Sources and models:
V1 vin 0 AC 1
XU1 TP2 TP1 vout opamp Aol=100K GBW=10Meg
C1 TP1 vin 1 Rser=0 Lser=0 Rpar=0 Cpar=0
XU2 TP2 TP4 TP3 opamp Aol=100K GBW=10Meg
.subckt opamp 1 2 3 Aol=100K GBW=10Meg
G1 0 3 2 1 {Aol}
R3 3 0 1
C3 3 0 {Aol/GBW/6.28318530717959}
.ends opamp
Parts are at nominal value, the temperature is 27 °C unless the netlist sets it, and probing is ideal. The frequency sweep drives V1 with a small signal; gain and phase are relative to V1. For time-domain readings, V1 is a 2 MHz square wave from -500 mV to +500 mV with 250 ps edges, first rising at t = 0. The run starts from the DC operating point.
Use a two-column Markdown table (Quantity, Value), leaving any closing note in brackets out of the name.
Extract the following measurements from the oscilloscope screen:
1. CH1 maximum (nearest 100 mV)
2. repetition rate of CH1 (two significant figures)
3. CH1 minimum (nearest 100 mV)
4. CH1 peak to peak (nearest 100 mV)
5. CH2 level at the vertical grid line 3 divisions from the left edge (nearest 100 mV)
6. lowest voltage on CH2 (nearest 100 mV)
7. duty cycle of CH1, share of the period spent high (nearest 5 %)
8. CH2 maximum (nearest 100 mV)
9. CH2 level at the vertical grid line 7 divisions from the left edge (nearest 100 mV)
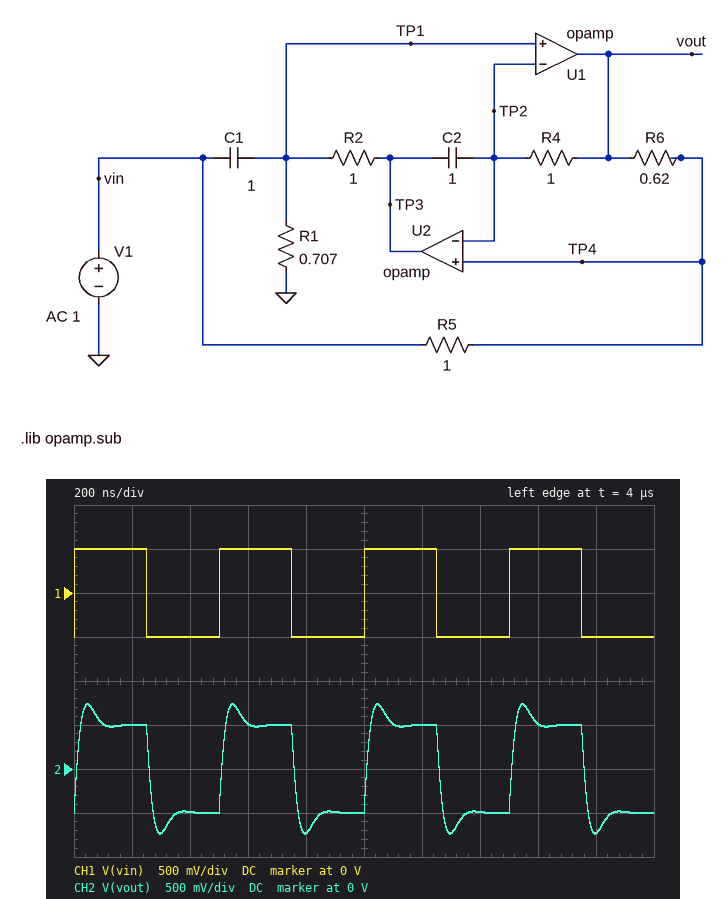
| Quantity | Value |
|---|---|
| CH1 maximum | 500 mV |
| repetition rate of CH1 | 2.0 MHz |
| CH1 minimum | -500 mV |
| CH1 peak to peak | 1.0 V |
| CH2 level at the vertical grid line 3 divisions from the left edge | 500 mV |
| lowest voltage on CH2 | -700 mV |
| duty cycle of CH1, share of the period spent high | 50 % |
| CH2 maximum | 700 mV |
| CH2 level at the vertical grid line 7 divisions from the left edge | -500 mV |
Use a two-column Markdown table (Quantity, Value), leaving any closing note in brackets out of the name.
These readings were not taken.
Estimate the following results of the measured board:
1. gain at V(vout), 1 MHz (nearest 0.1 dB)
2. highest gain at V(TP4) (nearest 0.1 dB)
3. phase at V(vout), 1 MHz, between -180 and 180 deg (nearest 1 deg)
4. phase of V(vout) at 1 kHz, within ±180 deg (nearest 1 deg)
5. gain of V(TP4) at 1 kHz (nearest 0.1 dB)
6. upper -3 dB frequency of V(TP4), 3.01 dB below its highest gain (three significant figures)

| Quantity | Value |
|---|---|
| gain at V(vout), 1 MHz | 0.1 dB |
| highest gain at V(TP4) | 1.4 dB |
| phase at V(vout), 1 MHz, between -180 and 180 deg | 0 deg |
| phase of V(vout) at 1 kHz, within ±180 deg | 0 deg |
| gain of V(TP4) at 1 kHz | 0 dB |
| upper -3 dB frequency of V(TP4), 3.01 dB below its highest gain | 11.9 MHz |
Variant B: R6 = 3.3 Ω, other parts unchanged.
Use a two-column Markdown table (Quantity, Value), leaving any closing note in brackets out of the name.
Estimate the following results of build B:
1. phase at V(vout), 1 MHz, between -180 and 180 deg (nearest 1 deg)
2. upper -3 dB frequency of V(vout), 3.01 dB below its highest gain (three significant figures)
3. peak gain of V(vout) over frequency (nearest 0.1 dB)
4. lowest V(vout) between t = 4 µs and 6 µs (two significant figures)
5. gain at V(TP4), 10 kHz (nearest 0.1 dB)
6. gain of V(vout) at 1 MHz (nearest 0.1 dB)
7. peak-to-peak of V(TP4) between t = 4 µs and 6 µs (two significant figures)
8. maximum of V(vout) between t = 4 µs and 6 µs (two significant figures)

| Quantity | Value |
|---|---|
| phase at V(vout), 1 MHz, between -180 and 180 deg | -1 deg |
| upper -3 dB frequency of V(vout), 3.01 dB below its highest gain | 439 mHz |
| peak gain of V(vout) over frequency | 10.4 dB |
| lowest V(vout) between t = 4 µs and 6 µs | -630 mV |
| gain at V(TP4), 10 kHz | 0 dB |
| gain of V(vout) at 1 MHz | 0.3 dB |
| peak-to-peak of V(TP4) between t = 4 µs and 6 µs | 1.1 V |
| maximum of V(vout) between t = 4 µs and 6 µs | 630 mV |
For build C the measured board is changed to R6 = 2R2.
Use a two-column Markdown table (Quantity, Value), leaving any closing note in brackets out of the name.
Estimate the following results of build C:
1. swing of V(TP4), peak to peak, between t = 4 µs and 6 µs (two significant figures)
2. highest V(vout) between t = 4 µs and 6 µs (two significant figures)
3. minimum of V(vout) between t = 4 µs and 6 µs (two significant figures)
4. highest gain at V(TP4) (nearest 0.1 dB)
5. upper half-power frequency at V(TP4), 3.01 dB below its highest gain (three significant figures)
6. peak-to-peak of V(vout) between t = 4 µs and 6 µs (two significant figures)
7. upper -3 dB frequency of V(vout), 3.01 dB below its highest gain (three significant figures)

| Quantity | Value |
|---|---|
| swing of V(TP4), peak to peak, between t = 4 µs and 6 µs | 1.1 V |
| highest V(vout) between t = 4 µs and 6 µs | 660 mV |
| minimum of V(vout) between t = 4 µs and 6 µs | -660 mV |
| highest gain at V(TP4) | 0.4 dB |
| upper half-power frequency at V(TP4), 3.01 dB below its highest gain | 21.9 MHz |
| peak-to-peak of V(vout) between t = 4 µs and 6 µs | 1.3 V |
| upper -3 dB frequency of V(vout), 3.01 dB below its highest gain | 425 mHz |
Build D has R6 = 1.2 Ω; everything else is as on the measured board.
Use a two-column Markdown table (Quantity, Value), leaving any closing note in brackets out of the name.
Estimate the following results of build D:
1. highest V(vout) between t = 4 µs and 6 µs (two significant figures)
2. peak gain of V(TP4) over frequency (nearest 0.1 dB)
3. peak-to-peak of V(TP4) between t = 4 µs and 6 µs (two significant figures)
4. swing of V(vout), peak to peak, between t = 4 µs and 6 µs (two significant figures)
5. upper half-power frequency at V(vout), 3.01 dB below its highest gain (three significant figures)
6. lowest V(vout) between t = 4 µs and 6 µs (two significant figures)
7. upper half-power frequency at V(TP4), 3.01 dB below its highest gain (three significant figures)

| Quantity | Value |
|---|---|
| highest V(vout) between t = 4 µs and 6 µs | 700 mV |
| peak gain of V(TP4) over frequency | 0.8 dB |
| peak-to-peak of V(TP4) between t = 4 µs and 6 µs | 1.2 V |
| swing of V(vout), peak to peak, between t = 4 µs and 6 µs | 1.4 V |
| upper half-power frequency at V(vout), 3.01 dB below its highest gain | 11.1 MHz |
| lowest V(vout) between t = 4 µs and 6 µs | -700 mV |
| upper half-power frequency at V(TP4), 3.01 dB below its highest gain | 12.8 MHz |
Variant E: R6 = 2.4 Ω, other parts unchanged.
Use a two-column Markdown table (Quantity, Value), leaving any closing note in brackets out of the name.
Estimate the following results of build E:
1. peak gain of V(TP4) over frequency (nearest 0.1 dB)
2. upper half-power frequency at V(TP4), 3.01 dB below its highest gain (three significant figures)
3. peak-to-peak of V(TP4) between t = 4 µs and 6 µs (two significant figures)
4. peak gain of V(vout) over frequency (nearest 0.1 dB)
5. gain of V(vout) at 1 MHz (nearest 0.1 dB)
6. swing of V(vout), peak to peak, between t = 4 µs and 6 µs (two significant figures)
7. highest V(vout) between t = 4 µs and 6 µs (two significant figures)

| Quantity | Value |
|---|---|
| peak gain of V(TP4) over frequency | 0.4 dB |
| upper half-power frequency at V(TP4), 3.01 dB below its highest gain | 27.9 MHz |
| peak-to-peak of V(TP4) between t = 4 µs and 6 µs | 1.1 V |
| peak gain of V(vout) over frequency | 7.6 dB |
| gain of V(vout) at 1 MHz | 0.3 dB |
| swing of V(vout), peak to peak, between t = 4 µs and 6 µs | 1.3 V |
| highest V(vout) between t = 4 µs and 6 µs | 650 mV |
